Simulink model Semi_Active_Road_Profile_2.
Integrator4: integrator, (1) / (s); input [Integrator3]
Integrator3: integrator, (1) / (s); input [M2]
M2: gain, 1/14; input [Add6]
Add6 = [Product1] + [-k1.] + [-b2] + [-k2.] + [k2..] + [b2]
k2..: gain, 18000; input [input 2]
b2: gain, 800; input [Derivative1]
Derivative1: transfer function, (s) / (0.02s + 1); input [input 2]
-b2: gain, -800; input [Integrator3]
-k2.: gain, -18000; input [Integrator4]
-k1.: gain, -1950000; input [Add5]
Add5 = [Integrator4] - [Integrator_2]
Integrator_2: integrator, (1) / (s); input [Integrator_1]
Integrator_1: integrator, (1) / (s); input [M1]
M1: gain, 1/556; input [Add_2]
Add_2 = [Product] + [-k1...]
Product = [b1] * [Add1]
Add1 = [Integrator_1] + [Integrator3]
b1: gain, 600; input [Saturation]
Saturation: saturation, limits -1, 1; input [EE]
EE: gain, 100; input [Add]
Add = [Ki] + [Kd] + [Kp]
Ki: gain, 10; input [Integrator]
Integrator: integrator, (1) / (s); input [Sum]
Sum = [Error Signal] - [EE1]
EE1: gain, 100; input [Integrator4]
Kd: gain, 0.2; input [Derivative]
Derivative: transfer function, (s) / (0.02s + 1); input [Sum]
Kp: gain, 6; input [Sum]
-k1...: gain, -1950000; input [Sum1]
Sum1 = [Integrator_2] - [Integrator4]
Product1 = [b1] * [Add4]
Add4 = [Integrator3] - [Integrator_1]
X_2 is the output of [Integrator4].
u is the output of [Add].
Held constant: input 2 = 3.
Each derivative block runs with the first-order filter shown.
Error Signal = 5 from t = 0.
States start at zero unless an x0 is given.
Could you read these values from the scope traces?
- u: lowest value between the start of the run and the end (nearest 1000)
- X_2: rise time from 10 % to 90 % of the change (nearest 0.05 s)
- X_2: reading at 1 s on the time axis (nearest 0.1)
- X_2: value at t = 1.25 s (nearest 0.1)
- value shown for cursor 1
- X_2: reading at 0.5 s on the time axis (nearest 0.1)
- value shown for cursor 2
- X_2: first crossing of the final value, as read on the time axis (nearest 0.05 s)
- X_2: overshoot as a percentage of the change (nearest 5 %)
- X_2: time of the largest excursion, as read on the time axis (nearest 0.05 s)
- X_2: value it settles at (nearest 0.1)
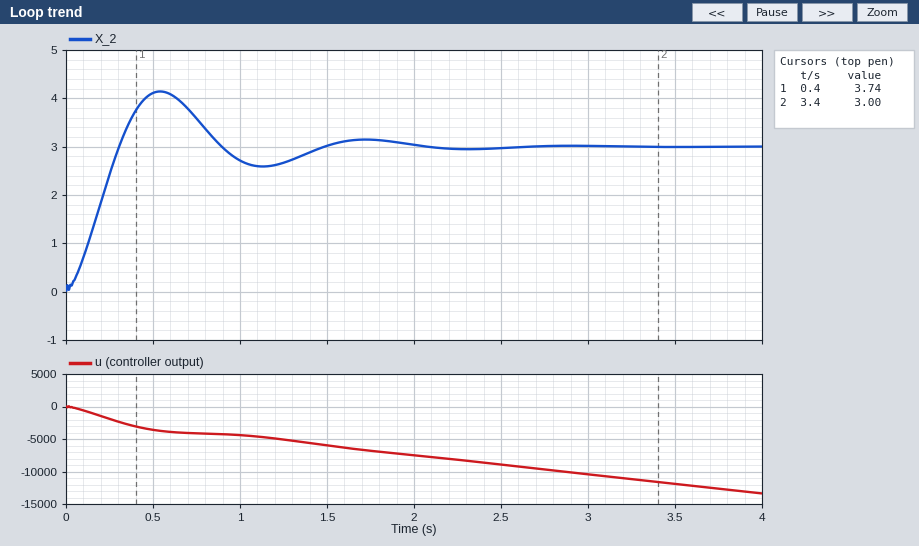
-13000
0.20 s
2.7
2.7
3.74
4.1
3.00
0.30 s
40 %
0.55 s
3.0
